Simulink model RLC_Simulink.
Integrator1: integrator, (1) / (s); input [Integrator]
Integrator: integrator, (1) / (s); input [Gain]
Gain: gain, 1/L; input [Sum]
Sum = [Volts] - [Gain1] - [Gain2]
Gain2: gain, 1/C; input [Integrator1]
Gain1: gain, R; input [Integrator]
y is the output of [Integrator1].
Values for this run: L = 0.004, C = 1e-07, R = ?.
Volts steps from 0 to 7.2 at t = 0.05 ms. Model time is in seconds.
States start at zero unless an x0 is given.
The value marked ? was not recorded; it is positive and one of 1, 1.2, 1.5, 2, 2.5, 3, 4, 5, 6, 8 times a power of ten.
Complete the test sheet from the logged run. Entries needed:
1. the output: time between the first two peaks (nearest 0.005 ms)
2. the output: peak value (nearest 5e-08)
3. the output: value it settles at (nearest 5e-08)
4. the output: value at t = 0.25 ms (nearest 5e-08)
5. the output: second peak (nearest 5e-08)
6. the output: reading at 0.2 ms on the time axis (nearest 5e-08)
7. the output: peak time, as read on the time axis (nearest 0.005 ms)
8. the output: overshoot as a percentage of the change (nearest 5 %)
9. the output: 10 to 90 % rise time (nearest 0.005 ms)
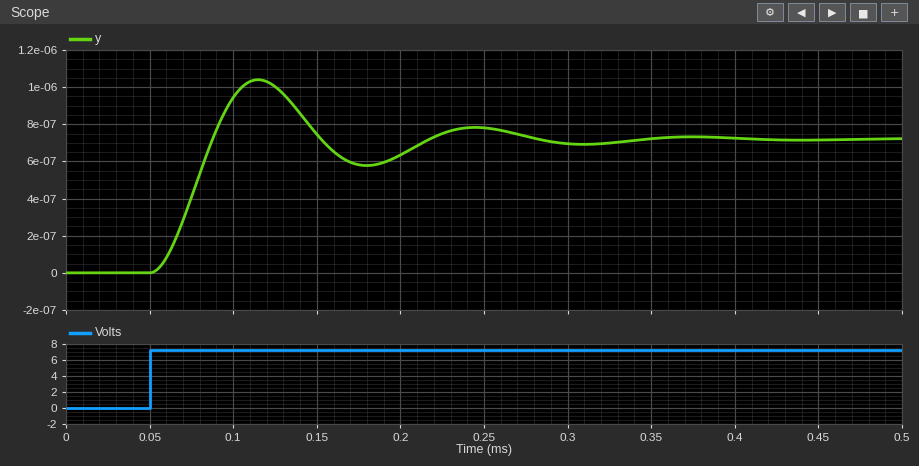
0.130 ms
0.00000105
0.00000070
0.00000080
0.00000080
0.00000065
0.115 ms
45 %
0.025 ms
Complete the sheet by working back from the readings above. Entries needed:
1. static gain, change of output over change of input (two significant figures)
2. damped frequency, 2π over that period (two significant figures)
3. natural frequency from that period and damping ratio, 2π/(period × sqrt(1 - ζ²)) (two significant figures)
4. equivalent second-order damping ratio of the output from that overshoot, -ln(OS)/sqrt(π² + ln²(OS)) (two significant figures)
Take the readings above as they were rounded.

0.000000097
48 rad/ms
50 rad/ms
0.25
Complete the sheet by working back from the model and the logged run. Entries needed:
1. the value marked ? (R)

100
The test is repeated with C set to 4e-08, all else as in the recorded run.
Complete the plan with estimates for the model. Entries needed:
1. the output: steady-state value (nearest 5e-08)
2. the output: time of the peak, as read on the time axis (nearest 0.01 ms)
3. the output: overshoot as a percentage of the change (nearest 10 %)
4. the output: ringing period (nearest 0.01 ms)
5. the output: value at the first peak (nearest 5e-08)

0.00000030
0.09 ms
60 %
0.08 ms
0.00000045
